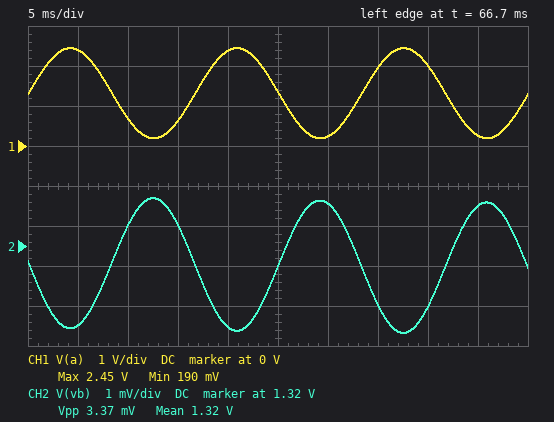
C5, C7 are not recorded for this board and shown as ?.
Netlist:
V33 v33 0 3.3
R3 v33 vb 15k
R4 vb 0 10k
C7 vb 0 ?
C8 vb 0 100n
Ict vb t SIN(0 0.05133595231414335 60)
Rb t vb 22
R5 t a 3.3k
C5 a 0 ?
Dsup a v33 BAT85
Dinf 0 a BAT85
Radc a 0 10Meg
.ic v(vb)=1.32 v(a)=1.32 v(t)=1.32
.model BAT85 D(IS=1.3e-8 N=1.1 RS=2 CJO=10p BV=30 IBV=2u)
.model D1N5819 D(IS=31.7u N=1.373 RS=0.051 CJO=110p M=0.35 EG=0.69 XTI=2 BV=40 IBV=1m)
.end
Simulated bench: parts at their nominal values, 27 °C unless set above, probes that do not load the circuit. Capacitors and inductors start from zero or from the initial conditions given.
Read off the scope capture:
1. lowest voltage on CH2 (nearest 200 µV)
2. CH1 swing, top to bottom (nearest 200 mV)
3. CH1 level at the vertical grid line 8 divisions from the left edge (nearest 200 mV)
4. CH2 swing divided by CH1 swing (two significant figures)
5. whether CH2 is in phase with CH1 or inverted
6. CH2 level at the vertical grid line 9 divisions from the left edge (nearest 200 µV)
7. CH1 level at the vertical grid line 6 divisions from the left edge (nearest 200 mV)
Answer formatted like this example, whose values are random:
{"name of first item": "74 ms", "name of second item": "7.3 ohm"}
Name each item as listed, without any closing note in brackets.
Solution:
{"lowest voltage on CH2": "1.3178 V", "CH1 swing, top to bottom": "2.2 V", "CH1 level at the vertical grid line 8 divisions from the left edge": "2.0 V", "CH2 swing divided by CH1 swing": "0.0015", "whether CH2 is in phase with CH1 or inverted": "inverted", "CH2 level at the vertical grid line 9 divisions from the left edge": "1.3210 V", "CH1 level at the vertical grid line 6 divisions from the left edge": "200 mV"}
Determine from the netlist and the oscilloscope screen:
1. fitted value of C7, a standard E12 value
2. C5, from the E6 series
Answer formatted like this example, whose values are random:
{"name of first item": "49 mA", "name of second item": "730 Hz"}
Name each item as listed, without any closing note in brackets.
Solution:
{"fitted value of C7, a standard E12 value": "15 µF", "C5, from the E6 series": "22 nF"}
